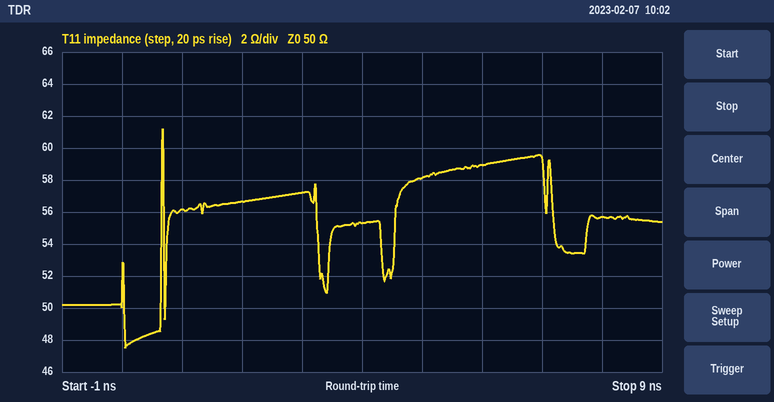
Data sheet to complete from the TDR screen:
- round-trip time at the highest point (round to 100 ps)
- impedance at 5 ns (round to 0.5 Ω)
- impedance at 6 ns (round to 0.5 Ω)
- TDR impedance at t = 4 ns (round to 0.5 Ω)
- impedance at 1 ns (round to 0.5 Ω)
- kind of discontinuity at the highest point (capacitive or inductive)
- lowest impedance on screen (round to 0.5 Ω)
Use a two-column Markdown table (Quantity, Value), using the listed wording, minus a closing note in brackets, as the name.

| Quantity | Value |
|---|---|
| round-trip time at the highest point | 700 ps |
| impedance at 5 ns | 58.0 Ω |
| impedance at 6 ns | 59.0 Ω |
| TDR impedance at t = 4 ns | 55.5 Ω |
| impedance at 1 ns | 56.0 Ω |
| kind of discontinuity at the highest point | inductive |
| lowest impedance on screen | 47.5 Ω |
